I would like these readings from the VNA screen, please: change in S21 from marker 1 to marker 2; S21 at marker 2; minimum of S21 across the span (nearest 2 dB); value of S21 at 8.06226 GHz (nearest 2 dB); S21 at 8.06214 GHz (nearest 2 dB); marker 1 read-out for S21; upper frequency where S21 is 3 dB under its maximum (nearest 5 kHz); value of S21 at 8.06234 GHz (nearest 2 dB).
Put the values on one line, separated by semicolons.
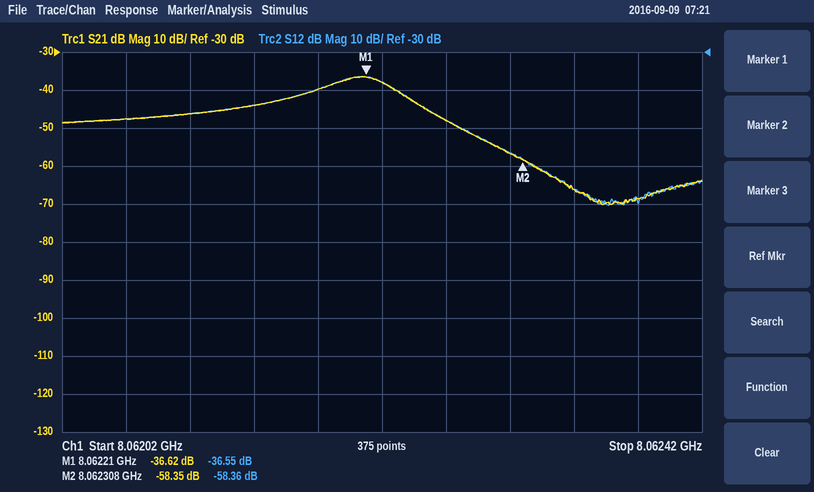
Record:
-21.73 dB; -58.35 dB; -70 dB; -48 dB; -44 dB; -36.62 dB; 8.062225 GHz; -66 dB
